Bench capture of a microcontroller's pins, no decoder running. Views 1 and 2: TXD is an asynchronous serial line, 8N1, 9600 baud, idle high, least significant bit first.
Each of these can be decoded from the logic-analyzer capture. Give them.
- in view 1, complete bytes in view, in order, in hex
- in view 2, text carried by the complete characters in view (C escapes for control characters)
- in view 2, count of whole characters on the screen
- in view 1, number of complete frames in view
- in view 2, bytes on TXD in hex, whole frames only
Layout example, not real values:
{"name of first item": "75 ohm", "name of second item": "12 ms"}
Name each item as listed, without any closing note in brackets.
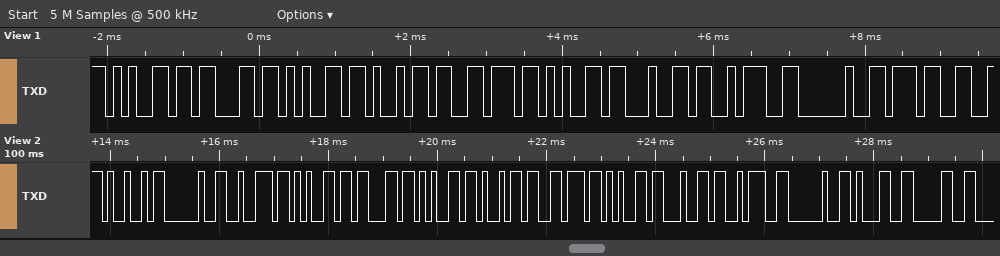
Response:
{"in view 1, complete bytes in view, in order, in hex": "65 63 65 69 76 65 64 3A 20 37", "in view 2, text carried by the complete characters in view": "\"I received: 10\"", "in view 2, count of whole characters on the screen": "14", "in view 1, number of complete frames in view": "10", "in view 2, bytes on TXD in hex, whole frames only": "0x49 0x20 0x72 0x65 0x63 0x65 0x69 0x76 0x65 0x64 0x3A 0x20 0x31 0x30"}
